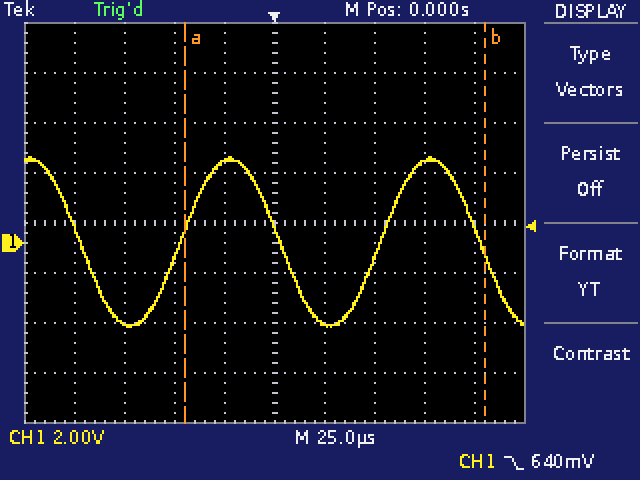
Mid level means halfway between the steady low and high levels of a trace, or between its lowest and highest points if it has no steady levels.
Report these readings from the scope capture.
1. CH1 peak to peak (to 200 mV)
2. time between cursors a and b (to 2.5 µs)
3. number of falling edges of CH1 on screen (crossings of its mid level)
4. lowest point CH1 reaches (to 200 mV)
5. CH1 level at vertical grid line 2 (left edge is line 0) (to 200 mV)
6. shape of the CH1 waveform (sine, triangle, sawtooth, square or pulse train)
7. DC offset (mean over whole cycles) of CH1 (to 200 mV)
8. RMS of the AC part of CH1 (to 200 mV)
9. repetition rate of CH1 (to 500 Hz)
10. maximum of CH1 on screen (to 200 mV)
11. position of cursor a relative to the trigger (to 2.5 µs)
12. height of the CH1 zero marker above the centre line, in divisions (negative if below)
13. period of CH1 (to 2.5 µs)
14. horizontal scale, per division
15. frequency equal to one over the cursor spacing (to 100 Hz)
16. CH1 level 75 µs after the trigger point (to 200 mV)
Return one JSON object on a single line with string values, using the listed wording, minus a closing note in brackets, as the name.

{"CH1 peak to peak": "6.8 V", "time between cursors a and b": "150.0 µs", "number of falling edges of CH1 on screen": "3", "lowest point CH1 reaches": "-3.4 V", "CH1 level at vertical grid line 2 (left edge is line 0)": "-3.2 V", "shape of the CH1 waveform": "sine", "DC offset (mean over whole cycles) of CH1": "0.0 V", "RMS of the AC part of CH1": "2.4 V", "repetition rate of CH1": "10.0 kHz", "maximum of CH1 on screen": "3.4 V", "position of cursor a relative to the trigger": "-45.0 µs", "height of the CH1 zero marker above the centre line, in divisions": "-0.4 div", "period of CH1": "100.0 µs", "horizontal scale, per division": "25 µs", "frequency equal to one over the cursor spacing": "6.7 kHz", "CH1 level 75 µs after the trigger point": "3.2 V"}
